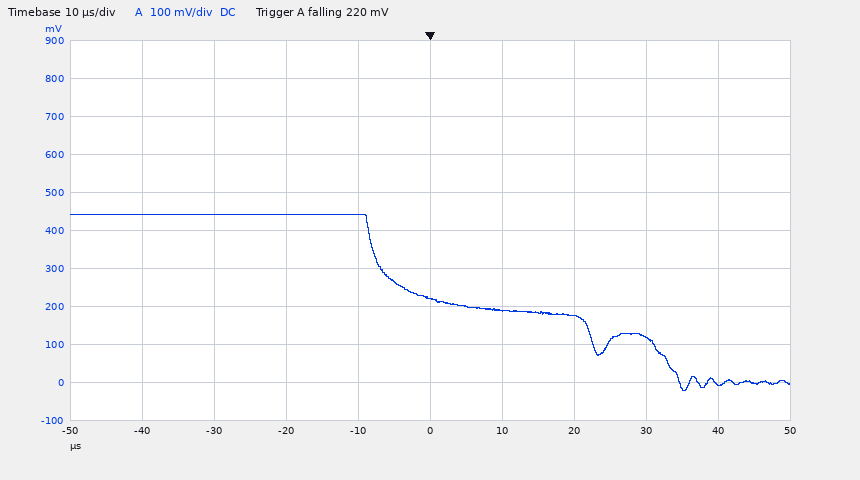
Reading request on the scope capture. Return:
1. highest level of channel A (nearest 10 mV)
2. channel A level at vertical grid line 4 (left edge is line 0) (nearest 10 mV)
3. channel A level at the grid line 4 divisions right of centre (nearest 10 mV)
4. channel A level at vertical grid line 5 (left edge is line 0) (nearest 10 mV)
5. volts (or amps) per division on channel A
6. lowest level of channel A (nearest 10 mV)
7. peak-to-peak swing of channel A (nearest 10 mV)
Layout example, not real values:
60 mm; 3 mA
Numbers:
440 mV; 440 mV; 0 mV; 220 mV; 100 mV; -20 mV; 460 mV
